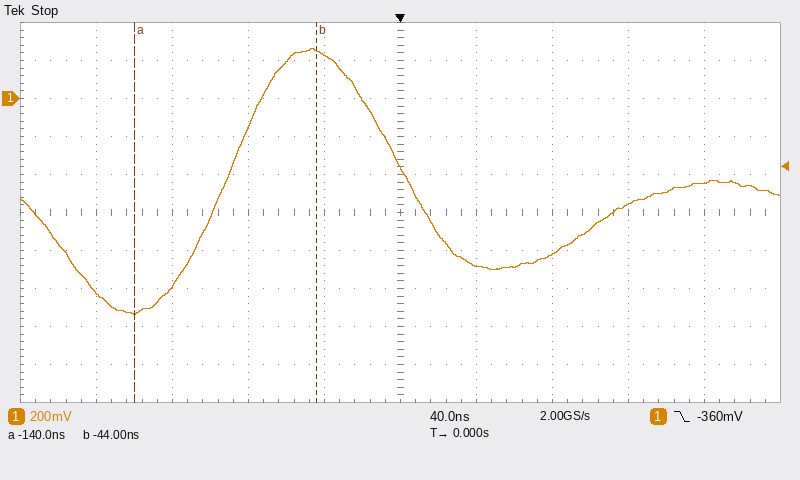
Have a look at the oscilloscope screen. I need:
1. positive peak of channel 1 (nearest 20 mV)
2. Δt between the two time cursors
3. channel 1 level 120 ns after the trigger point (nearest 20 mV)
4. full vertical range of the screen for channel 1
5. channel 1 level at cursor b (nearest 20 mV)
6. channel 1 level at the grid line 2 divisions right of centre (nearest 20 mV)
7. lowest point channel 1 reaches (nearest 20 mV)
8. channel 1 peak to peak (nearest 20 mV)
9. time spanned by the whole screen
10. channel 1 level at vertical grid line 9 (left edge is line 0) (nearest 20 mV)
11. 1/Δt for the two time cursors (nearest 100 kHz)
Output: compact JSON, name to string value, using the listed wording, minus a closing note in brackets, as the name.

{"positive peak of channel 1": "260 mV", "Δt between the two time cursors": "96 ns", "channel 1 level 120 ns after the trigger point": "-560 mV", "full vertical range of the screen for channel 1": "2 V", "channel 1 level at cursor b": "260 mV", "channel 1 level at the grid line 2 divisions right of centre": "-820 mV", "lowest point channel 1 reaches": "-1.14 V", "channel 1 peak to peak": "1.40 V", "time spanned by the whole screen": "400 ns", "channel 1 level at vertical grid line 9 (left edge is line 0)": "-440 mV", "1/Δt for the two time cursors": "10.4 MHz"}
